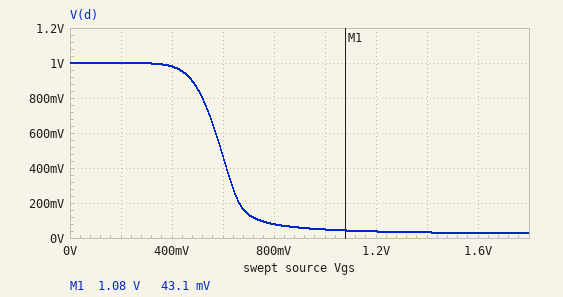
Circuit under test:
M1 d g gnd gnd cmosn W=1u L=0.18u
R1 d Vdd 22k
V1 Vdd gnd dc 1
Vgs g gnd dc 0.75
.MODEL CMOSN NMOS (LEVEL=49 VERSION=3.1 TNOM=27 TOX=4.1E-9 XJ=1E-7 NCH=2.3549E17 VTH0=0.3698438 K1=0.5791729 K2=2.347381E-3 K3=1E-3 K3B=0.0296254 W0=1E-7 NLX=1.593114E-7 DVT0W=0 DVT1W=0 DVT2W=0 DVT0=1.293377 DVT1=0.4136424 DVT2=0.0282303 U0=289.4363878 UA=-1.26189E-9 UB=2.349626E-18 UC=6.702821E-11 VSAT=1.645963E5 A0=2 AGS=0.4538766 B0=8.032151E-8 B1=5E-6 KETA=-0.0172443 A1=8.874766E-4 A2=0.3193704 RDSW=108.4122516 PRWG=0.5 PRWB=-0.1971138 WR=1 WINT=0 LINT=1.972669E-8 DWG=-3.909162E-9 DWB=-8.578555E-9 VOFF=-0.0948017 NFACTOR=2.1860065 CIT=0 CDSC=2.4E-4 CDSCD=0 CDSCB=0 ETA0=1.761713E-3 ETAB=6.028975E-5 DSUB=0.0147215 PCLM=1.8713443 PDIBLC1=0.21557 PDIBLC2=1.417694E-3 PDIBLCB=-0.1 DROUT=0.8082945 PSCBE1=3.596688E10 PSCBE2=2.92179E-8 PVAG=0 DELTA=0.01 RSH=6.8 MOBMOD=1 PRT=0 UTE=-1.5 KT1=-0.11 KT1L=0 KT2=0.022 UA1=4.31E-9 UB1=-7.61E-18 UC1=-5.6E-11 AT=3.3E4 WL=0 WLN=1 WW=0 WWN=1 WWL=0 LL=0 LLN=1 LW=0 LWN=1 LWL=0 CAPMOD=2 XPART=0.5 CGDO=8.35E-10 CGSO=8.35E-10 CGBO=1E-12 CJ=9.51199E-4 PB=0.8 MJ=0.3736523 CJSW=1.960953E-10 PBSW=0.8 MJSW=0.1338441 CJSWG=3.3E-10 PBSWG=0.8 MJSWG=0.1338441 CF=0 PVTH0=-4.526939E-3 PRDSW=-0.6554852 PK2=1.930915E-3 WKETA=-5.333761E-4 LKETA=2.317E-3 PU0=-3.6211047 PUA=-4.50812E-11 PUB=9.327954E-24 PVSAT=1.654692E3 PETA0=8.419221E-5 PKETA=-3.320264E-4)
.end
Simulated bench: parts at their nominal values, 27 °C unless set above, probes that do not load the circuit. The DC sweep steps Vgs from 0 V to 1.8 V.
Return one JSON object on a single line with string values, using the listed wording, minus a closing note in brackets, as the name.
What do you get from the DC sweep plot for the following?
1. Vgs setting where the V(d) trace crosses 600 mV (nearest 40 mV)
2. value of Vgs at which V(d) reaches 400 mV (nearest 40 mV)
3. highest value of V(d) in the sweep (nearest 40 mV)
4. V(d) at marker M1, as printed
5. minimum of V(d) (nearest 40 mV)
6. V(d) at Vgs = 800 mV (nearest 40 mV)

{"Vgs setting where the V(d) trace crosses 600 mV": "560 mV", "value of Vgs at which V(d) reaches 400 mV": "600 mV", "highest value of V(d) in the sweep": "1.00 V", "V(d) at marker M1, as printed": "43.1 mV", "minimum of V(d)": "40 mV", "V(d) at Vgs = 800 mV": "80 mV"}
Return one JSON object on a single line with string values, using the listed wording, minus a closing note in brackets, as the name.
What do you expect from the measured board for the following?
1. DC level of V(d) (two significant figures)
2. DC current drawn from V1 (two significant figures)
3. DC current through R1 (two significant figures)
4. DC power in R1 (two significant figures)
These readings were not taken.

{"DC level of V(d)": "98 mV", "DC current drawn from V1": "41 µA", "DC current through R1": "41 µA", "DC power in R1": "37 µW"}
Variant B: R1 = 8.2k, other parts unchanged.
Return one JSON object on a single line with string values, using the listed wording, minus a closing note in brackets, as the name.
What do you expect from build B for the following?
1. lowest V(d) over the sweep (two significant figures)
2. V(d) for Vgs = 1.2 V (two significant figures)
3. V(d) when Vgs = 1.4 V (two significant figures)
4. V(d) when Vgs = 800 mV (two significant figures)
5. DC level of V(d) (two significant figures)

{"lowest V(d) over the sweep": "71 mV", "V(d) for Vgs = 1.2 V": "100 mV", "V(d) when Vgs = 1.4 V": "85 mV", "V(d) when Vgs = 800 mV": "280 mV", "DC level of V(d)": "390 mV"}
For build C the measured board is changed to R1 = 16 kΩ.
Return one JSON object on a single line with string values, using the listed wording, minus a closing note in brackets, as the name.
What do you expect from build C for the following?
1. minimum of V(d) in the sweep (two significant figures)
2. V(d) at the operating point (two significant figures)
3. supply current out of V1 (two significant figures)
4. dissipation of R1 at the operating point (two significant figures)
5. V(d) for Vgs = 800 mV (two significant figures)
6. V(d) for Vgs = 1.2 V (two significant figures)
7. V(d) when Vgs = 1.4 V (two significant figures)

{"minimum of V(d) in the sweep": "37 mV", "V(d) at the operating point": "150 mV", "supply current out of V1": "53 µA", "dissipation of R1 at the operating point": "46 µW", "V(d) for Vgs = 800 mV": "110 mV", "V(d) for Vgs = 1.2 V": "52 mV", "V(d) when Vgs = 1.4 V": "44 mV"}
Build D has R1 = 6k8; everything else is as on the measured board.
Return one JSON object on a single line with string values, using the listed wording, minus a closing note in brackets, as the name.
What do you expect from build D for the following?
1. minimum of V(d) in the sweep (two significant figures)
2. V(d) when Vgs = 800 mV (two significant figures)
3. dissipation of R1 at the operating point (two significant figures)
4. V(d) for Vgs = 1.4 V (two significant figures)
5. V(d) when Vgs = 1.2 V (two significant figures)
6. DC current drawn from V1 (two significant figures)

{"minimum of V(d) in the sweep": "85 mV", "V(d) when Vgs = 800 mV": "370 mV", "dissipation of R1 at the operating point": "41 µW", "V(d) for Vgs = 1.4 V": "100 mV", "V(d) when Vgs = 1.2 V": "120 mV", "DC current drawn from V1": "77 µA"}
